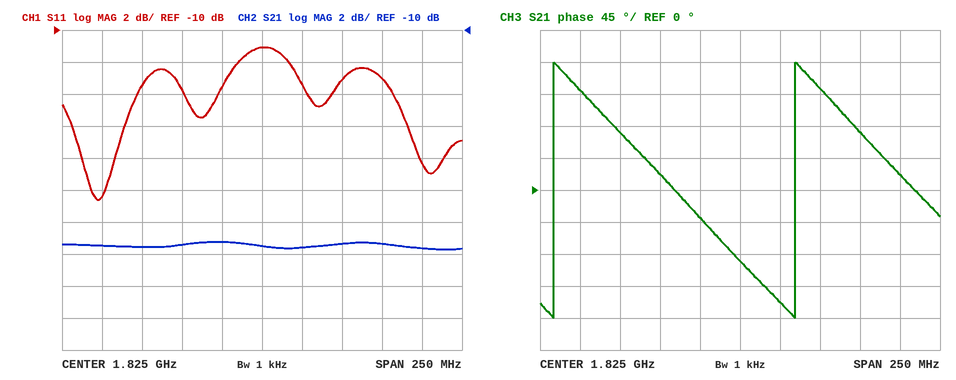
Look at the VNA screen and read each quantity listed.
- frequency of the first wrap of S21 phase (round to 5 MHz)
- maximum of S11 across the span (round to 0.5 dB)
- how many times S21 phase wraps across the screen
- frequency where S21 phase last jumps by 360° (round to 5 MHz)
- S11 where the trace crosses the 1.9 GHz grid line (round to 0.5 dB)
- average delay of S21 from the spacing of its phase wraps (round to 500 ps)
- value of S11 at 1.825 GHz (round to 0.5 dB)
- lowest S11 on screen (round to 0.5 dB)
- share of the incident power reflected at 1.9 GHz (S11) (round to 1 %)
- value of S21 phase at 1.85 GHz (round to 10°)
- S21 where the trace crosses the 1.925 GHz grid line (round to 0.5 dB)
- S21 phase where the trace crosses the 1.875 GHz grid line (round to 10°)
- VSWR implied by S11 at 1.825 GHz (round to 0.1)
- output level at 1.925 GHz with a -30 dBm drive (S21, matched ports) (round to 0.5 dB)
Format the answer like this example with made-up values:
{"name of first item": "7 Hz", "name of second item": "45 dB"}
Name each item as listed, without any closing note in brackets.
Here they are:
{"frequency of the first wrap of S21 phase": "1.710 GHz", "maximum of S11 across the span": "-11.0 dB", "how many times S21 phase wraps across the screen": "2", "frequency where S21 phase last jumps by 360°": "1.860 GHz", "S11 where the trace crosses the 1.9 GHz grid line": "-13.0 dB", "average delay of S21 from the spacing of its phase wraps": "6.5 ns", "value of S11 at 1.825 GHz": "-11.0 dB", "lowest S11 on screen": "-20.5 dB", "share of the incident power reflected at 1.9 GHz (S11)": "5 %", "value of S21 phase at 1.85 GHz": "-160°", "S21 where the trace crosses the 1.925 GHz grid line": "-23.5 dB", "S21 phase where the trace crosses the 1.875 GHz grid line": "140°", "VSWR implied by S11 at 1.825 GHz": "1.8", "output level at 1.925 GHz with a -30 dBm drive (S21, matched ports)": "-53.5 dBm"}
